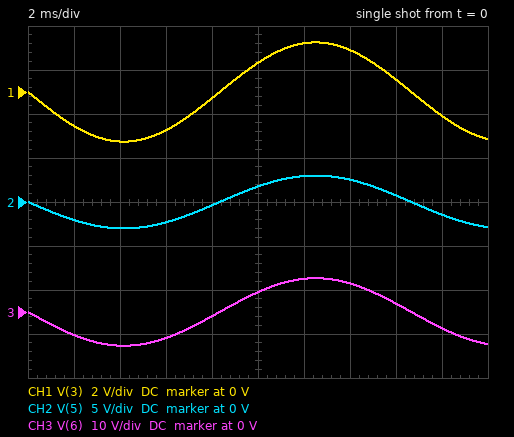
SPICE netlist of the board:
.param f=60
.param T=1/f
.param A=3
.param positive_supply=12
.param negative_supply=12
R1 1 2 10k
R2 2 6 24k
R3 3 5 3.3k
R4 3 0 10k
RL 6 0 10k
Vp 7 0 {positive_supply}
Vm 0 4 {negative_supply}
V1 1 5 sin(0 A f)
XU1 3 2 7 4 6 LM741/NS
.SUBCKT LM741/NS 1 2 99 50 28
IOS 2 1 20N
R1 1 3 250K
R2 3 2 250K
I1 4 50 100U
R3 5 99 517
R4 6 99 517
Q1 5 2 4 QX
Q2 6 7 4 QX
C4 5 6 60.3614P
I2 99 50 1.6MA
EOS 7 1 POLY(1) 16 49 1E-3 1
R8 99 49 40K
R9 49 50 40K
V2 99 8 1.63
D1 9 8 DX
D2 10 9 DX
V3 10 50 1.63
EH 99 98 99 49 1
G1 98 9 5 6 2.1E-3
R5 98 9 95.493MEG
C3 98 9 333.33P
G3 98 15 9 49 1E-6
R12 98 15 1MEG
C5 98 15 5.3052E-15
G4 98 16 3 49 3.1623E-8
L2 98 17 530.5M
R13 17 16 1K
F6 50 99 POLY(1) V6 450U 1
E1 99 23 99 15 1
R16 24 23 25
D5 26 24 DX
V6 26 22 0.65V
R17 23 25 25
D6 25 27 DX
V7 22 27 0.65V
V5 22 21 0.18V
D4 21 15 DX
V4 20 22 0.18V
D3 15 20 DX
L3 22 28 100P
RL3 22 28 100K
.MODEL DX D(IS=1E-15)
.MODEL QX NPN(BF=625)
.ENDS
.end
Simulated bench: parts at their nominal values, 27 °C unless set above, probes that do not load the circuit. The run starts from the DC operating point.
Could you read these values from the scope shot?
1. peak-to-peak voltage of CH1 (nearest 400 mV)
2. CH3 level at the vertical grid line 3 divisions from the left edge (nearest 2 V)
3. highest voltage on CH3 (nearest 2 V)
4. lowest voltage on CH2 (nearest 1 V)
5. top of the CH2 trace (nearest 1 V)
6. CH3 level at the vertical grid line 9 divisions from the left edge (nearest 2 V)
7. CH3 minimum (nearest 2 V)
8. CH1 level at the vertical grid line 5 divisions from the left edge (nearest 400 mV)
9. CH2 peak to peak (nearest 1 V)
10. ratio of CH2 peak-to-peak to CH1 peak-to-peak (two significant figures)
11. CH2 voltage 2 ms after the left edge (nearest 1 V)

4.4 V
-6 V
8 V
-3 V
3 V
-4 V
-8 V
1.2 V
6 V
1.3
-2 V
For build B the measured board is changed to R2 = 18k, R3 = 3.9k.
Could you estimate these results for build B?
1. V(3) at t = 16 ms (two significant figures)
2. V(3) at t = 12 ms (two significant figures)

540 mV
2.1 V
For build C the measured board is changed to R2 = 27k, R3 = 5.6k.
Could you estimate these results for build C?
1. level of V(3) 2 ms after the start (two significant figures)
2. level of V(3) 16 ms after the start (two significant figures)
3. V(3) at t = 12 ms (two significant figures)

-1.3 V
480 mV
1.9 V
